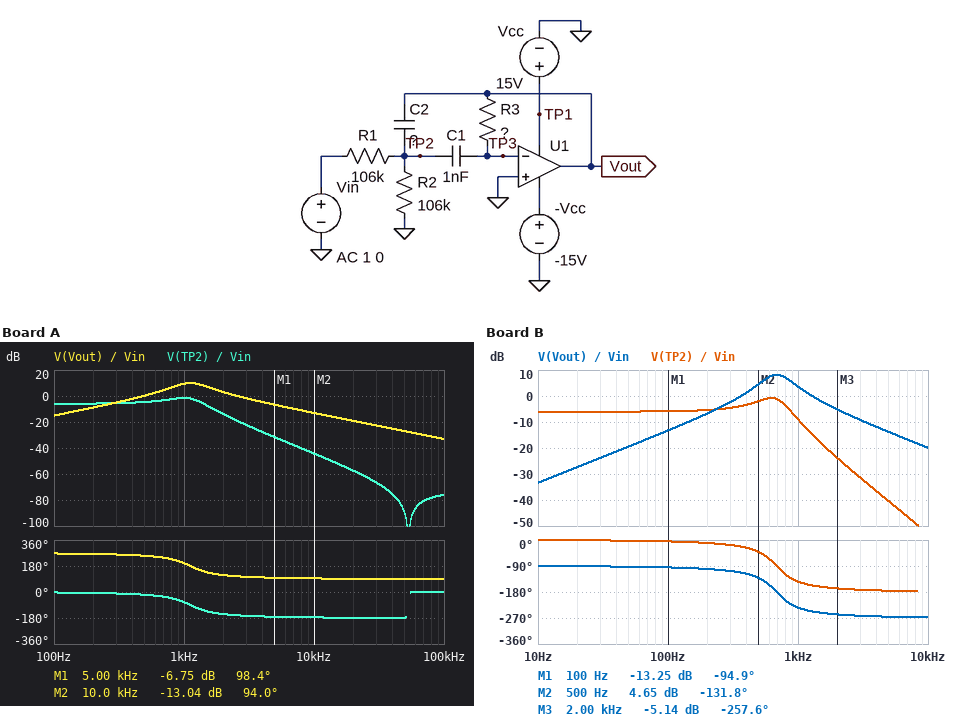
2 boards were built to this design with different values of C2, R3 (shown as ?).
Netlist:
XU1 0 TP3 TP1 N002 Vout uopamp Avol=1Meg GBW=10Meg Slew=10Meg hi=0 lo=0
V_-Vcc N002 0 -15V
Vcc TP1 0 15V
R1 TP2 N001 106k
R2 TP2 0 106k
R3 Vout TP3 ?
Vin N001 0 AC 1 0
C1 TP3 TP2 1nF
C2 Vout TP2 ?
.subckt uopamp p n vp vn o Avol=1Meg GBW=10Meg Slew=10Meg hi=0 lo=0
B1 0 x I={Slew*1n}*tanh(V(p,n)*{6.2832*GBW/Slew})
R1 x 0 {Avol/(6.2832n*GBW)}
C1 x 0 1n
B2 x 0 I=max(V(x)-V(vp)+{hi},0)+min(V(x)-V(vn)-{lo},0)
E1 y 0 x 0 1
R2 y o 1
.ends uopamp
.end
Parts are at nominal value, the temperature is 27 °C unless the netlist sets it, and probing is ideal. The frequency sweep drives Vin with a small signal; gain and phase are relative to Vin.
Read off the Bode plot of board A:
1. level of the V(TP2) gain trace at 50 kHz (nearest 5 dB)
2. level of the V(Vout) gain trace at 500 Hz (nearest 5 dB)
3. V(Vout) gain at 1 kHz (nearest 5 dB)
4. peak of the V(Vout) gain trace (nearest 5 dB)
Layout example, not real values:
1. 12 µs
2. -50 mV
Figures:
1. -90 dB
2. 0 dB
3. 10 dB
4. 10 dB
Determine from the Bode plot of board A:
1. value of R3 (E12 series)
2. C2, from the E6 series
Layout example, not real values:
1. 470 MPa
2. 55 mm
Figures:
1. 560 kΩ
2. 680 pF
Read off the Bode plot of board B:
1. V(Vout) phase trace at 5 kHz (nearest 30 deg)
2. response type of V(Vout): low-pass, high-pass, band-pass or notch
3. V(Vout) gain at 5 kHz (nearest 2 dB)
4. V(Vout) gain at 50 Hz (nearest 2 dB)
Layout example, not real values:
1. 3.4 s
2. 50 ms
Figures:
1. -270 deg
2. band-pass
3. -14 dB
4. -20 dB
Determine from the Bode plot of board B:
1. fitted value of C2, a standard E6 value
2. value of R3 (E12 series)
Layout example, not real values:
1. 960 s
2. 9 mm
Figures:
1. 1.5 nF
2. 680 kΩ
